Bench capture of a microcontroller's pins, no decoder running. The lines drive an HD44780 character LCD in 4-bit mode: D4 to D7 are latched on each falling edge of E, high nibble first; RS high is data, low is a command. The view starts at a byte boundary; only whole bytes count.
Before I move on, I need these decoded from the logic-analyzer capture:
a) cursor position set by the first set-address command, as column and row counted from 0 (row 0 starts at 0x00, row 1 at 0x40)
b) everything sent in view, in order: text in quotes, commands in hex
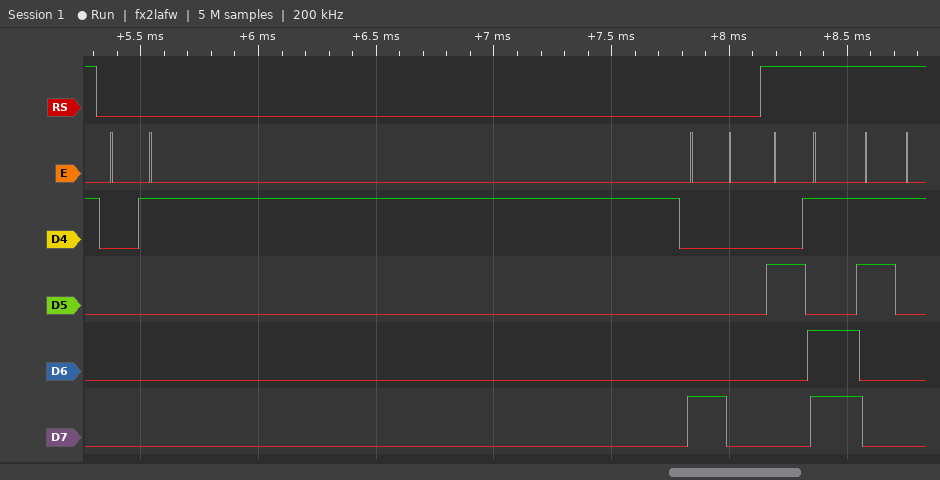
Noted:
column 0, row 0
0x01 0x80 "-1"
